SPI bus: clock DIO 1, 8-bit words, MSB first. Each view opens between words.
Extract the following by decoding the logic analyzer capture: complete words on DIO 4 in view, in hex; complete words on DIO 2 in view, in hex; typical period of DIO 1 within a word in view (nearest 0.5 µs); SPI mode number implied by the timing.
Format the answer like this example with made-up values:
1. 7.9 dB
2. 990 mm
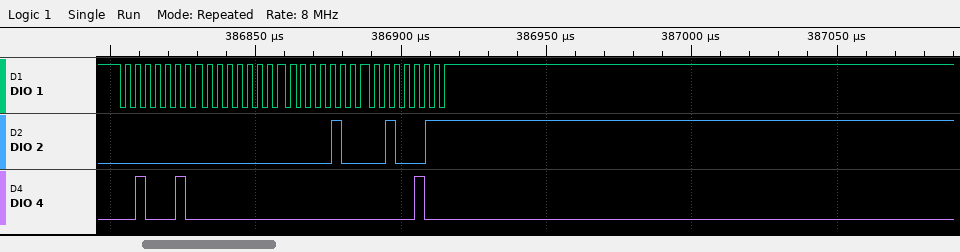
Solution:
1. 22, 00, 00, 04
2. 00, 00, 04, 23
3. 3.5 µs
4. 2
